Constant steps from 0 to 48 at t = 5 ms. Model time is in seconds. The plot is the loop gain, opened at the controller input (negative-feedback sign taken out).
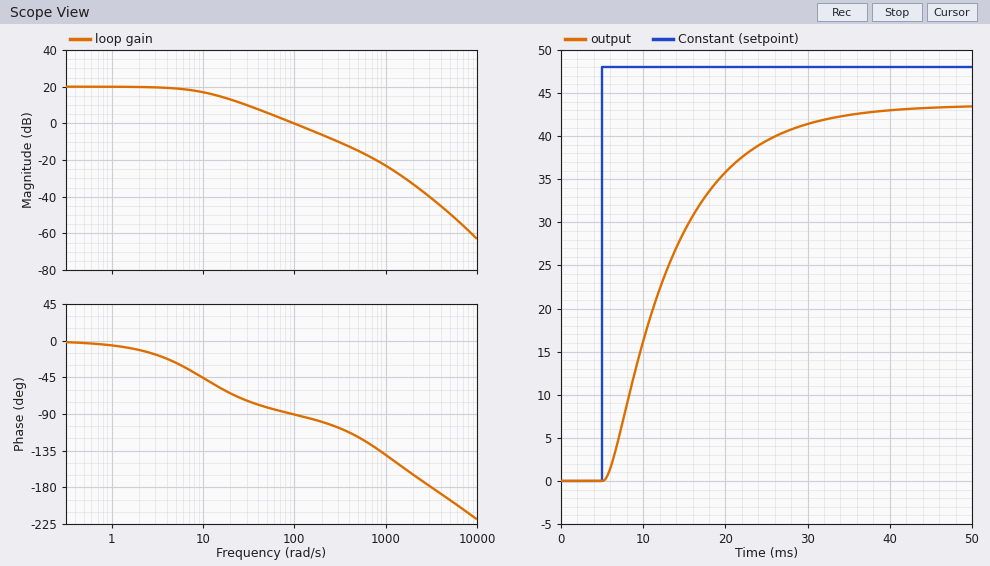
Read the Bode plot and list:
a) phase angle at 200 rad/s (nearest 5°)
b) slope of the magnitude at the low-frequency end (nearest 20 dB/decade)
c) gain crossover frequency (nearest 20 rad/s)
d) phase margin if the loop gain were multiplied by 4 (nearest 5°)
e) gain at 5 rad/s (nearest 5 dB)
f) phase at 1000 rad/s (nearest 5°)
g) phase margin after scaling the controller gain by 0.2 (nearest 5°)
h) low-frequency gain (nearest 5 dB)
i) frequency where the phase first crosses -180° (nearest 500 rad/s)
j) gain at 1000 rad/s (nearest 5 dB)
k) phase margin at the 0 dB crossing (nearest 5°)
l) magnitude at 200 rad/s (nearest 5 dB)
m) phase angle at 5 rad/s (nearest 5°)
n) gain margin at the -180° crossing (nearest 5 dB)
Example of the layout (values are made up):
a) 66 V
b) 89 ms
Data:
a) -100°
b) 0 dB/decade
c) 100 rad/s
d) 70°
e) 20 dB
f) -140°
g) 120°
h) 20 dB
i) 3000 rad/s
j) -25 dB
k) 90°
l) -5 dB
m) -25°
n) 40 dB
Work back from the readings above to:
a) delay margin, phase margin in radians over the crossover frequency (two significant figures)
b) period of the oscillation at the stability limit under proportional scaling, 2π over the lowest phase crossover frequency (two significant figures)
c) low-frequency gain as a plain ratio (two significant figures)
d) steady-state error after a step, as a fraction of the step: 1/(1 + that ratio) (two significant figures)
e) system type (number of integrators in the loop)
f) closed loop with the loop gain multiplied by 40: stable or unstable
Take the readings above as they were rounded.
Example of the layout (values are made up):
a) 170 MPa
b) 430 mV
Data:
a) 0.016 s
b) 0.0021 s
c) 10
d) 0.091
e) 0
f) stable
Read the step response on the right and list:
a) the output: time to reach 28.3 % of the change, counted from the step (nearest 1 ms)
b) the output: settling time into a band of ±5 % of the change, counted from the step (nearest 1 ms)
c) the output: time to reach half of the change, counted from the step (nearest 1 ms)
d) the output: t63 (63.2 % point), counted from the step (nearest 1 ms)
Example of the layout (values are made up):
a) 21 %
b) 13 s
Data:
a) 4 ms
b) 25 ms
c) 7 ms
d) 9 ms
